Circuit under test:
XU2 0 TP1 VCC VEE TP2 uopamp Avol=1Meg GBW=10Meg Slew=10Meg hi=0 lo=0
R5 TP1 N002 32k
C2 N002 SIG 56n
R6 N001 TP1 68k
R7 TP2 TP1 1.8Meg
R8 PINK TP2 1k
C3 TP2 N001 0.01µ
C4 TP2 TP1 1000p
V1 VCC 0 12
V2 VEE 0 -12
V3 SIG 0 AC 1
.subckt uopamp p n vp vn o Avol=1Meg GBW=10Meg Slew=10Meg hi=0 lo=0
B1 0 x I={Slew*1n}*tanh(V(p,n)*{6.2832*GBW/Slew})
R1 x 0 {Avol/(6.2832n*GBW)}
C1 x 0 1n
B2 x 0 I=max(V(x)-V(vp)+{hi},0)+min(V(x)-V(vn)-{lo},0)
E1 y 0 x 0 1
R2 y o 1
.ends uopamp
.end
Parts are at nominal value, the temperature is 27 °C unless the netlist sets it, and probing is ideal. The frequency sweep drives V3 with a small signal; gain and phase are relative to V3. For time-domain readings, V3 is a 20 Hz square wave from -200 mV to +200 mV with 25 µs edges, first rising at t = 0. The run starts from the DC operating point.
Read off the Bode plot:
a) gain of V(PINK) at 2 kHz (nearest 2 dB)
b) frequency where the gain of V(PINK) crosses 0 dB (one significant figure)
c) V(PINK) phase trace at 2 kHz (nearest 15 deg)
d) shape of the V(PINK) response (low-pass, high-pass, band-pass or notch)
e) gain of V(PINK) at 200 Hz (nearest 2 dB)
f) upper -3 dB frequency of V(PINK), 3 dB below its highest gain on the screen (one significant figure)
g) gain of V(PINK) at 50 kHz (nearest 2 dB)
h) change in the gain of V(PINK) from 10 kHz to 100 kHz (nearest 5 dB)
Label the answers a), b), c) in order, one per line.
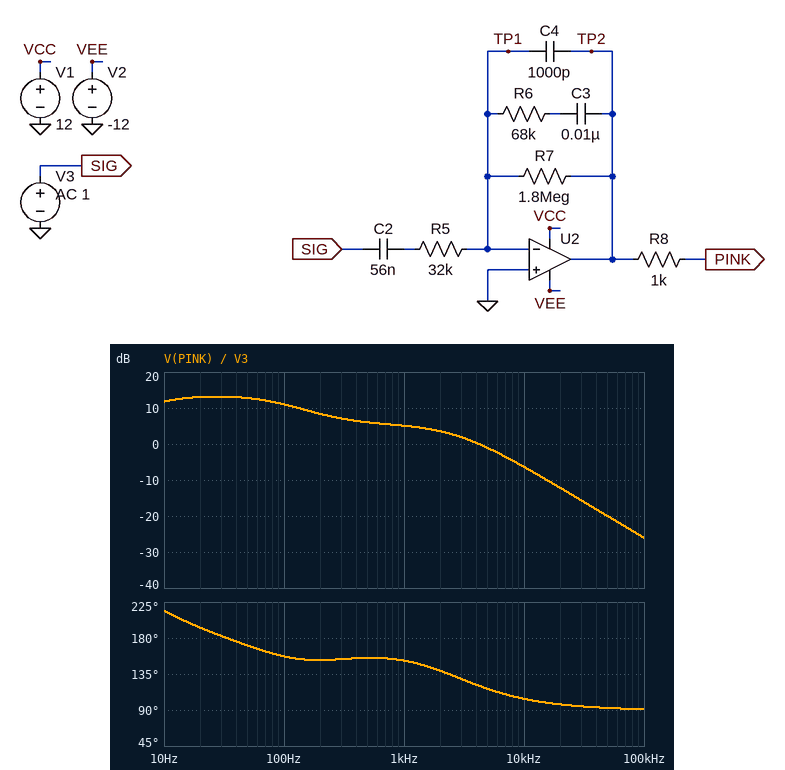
a) 4 dB
b) 4 kHz
c) 135 deg
d) low-pass
e) 8 dB
f) 100 Hz
g) -20 dB
h) -20 dB
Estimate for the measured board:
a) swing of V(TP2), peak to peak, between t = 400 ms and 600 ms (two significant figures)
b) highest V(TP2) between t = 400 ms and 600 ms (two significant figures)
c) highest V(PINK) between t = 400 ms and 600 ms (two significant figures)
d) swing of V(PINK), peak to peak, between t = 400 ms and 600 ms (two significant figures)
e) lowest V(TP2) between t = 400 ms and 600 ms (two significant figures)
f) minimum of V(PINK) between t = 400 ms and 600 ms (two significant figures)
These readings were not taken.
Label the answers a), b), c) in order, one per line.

a) 2.4 V
b) 1.2 V
c) 1.2 V
d) 2.4 V
e) -1.2 V
f) -1.2 V
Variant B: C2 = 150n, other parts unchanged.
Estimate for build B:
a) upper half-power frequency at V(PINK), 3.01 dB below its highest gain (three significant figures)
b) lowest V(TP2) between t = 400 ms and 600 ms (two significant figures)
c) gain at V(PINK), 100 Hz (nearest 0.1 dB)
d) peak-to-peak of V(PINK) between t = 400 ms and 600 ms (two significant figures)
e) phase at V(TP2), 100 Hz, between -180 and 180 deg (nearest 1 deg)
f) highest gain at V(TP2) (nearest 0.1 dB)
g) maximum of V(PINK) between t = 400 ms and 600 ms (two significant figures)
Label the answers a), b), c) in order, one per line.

a) 47.8 Hz
b) -2.4 V
c) 13.1 dB
d) 4.9 V
e) 134 deg
f) 20.6 dB
g) 2.4 V
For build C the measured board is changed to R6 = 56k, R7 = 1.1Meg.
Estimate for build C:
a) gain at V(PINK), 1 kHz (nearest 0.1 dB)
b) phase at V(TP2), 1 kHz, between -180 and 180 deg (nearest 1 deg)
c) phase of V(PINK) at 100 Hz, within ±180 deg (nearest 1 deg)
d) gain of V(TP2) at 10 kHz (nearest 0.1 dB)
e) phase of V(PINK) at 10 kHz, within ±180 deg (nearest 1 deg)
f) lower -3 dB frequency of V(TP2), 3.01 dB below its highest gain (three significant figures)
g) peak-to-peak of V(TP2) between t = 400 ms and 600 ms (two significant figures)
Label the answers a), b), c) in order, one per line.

a) 3.6 dB
b) 153 deg
c) 156 deg
d) -6.5 dB
e) 107 deg
f) 10.2 Hz
g) 2.5 V
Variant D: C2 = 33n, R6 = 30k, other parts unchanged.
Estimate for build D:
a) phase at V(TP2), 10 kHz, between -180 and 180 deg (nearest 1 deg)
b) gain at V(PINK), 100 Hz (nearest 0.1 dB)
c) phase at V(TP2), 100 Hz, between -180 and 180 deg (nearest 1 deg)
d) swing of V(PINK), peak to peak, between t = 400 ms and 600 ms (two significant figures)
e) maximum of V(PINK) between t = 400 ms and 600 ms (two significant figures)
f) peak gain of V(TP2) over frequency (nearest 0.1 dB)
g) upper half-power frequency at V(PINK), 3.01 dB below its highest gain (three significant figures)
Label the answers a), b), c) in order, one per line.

a) 118 deg
b) 8.0 dB
c) 161 deg
d) 1.5 V
e) 770 mV
f) 9.0 dB
g) 182 Hz
